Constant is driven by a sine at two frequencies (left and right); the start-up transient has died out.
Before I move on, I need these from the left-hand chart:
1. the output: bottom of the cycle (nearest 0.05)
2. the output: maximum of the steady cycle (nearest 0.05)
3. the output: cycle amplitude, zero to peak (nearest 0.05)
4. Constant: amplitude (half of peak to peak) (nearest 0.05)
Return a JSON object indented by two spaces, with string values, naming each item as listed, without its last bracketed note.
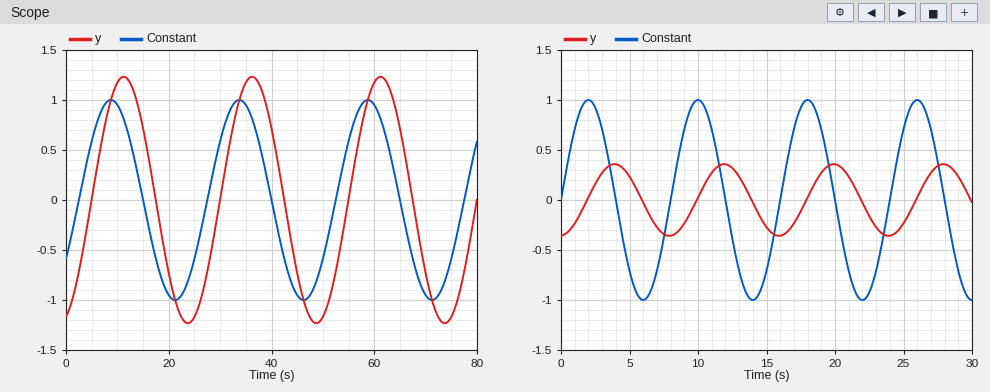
{
  "the output: bottom of the cycle": "-1.25",
  "the output: maximum of the steady cycle": "1.25",
  "the output: cycle amplitude, zero to peak": "1.25",
  "Constant: amplitude (half of peak to peak)": "1.00"
}
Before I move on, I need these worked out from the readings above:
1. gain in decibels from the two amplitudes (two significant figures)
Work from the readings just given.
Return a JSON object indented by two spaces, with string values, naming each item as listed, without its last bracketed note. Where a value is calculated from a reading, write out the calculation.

{
  "gain in decibels from the two amplitudes": "20 log10(1.25 / 1) = 1.9 dB"
}
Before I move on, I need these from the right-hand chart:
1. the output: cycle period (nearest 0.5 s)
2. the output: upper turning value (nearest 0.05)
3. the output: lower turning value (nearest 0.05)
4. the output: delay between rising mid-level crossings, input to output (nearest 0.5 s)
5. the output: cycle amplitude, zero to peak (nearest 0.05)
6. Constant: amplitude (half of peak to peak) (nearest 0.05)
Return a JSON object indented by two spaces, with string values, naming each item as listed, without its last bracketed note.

{
  "the output: cycle period": "8.0 s",
  "the output: upper turning value": "0.35",
  "the output: lower turning value": "-0.35",
  "the output: delay between rising mid-level crossings, input to output": "2.0 s",
  "the output: cycle amplitude, zero to peak": "0.35",
  "Constant: amplitude (half of peak to peak)": "1.00"
}
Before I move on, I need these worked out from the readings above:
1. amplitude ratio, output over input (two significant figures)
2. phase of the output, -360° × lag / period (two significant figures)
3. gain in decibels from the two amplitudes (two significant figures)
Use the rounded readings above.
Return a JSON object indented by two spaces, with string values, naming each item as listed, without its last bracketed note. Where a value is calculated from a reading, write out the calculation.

{
  "amplitude ratio, output over input": "0.35 / 1 = 0.35",
  "phase of the output, -360° × lag / period": "-360 × 2 / 8 = -90°",
  "gain in decibels from the two amplitudes": "20 log10(0.35 / 1) = -9.1 dB"
}
